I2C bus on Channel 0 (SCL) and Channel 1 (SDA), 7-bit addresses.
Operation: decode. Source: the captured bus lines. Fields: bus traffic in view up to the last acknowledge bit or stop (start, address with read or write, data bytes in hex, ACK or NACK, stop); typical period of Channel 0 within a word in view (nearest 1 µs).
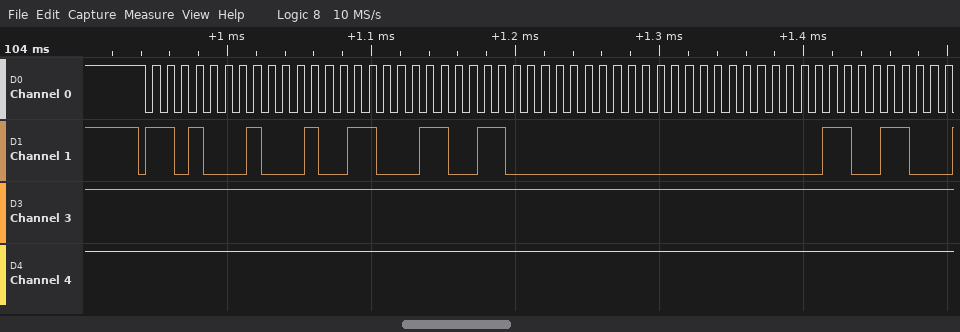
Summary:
start, address 68 read ACK, 26 ACK, 66 ACK, 00 ACK, 00 ACK, 33 ACK
10 µs
